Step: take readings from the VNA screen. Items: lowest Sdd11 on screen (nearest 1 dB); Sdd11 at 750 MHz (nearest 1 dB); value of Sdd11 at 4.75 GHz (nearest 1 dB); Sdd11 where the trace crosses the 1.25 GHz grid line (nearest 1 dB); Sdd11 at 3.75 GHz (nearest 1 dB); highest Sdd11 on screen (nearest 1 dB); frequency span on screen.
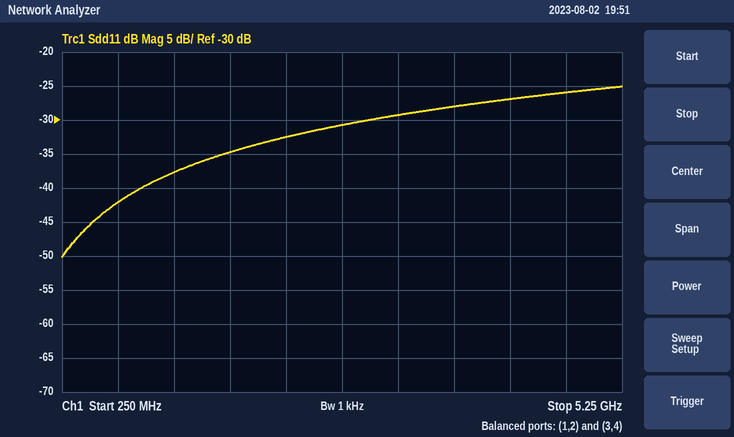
-50 dB
-42 dB
-26 dB
-38 dB
-28 dB
-25 dB
5 GHz
